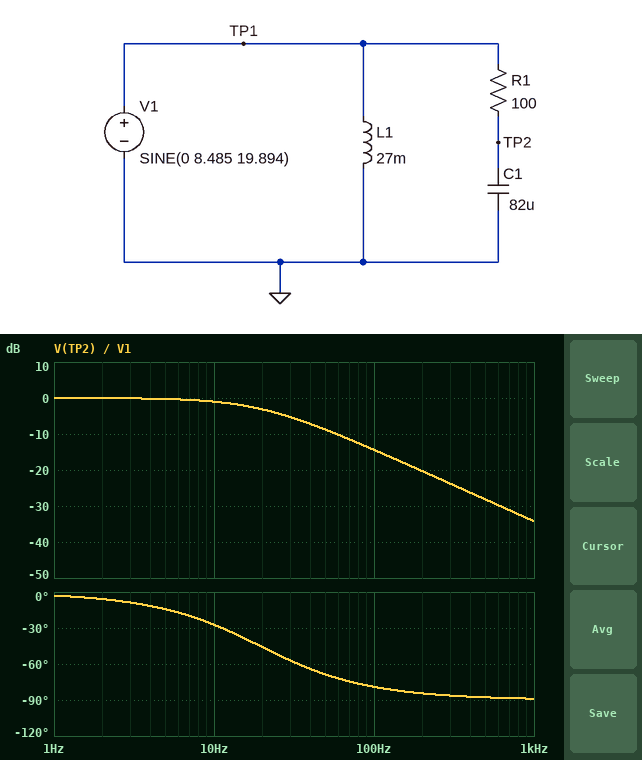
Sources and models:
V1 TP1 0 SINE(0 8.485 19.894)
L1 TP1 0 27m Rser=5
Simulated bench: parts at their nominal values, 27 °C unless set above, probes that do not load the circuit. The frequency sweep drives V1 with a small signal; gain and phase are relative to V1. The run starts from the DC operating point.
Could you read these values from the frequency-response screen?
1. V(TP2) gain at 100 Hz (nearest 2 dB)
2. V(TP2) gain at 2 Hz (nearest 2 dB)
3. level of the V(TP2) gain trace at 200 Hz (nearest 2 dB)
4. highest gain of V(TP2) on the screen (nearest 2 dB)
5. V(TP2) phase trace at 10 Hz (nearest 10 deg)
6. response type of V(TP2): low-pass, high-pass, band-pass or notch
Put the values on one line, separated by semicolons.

-14 dB; 0 dB; -20 dB; 0 dB; -30 deg; low-pass
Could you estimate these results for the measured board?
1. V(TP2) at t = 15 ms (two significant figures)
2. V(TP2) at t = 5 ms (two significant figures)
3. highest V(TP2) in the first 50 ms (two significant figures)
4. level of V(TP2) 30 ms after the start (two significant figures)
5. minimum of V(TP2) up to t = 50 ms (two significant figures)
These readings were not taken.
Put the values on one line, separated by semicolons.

5.9 V; 1.3 V; 6.4 V; 1.2 V; -5.9 V
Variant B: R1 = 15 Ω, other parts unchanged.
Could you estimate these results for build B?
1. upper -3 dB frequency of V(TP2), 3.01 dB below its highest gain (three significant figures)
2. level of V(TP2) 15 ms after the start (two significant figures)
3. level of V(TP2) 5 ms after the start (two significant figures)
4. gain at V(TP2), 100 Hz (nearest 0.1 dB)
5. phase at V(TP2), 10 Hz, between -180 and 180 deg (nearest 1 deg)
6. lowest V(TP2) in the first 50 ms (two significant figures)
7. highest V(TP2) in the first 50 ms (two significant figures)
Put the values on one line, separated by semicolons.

129 Hz; 8.3 V; 3.8 V; -2.0 dB; -4 deg; -8.4 V; 8.4 V
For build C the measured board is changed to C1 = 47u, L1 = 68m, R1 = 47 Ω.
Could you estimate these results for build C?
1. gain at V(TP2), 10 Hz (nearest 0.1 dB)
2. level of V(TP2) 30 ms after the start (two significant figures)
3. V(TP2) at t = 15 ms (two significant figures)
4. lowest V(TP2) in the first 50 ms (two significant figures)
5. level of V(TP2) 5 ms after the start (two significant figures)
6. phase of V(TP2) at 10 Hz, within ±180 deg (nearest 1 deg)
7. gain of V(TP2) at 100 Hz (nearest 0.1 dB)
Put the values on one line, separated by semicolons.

-0.1 dB; -2.7 V; 8.2 V; -8.2 V; 3.1 V; -8 deg; -4.7 dB
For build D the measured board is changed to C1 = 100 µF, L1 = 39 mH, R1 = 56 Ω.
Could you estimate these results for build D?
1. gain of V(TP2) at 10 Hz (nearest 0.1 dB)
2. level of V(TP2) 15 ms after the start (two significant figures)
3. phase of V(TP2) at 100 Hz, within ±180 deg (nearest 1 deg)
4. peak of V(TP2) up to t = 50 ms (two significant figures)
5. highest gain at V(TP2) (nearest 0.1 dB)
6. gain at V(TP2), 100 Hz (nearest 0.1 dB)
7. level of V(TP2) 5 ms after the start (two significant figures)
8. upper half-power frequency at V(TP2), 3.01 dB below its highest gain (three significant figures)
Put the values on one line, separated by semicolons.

-0.5 dB; 6.9 V; -74 deg; 7.1 V; 0 dB; -11.3 dB; 1.7 V; 28.4 Hz
